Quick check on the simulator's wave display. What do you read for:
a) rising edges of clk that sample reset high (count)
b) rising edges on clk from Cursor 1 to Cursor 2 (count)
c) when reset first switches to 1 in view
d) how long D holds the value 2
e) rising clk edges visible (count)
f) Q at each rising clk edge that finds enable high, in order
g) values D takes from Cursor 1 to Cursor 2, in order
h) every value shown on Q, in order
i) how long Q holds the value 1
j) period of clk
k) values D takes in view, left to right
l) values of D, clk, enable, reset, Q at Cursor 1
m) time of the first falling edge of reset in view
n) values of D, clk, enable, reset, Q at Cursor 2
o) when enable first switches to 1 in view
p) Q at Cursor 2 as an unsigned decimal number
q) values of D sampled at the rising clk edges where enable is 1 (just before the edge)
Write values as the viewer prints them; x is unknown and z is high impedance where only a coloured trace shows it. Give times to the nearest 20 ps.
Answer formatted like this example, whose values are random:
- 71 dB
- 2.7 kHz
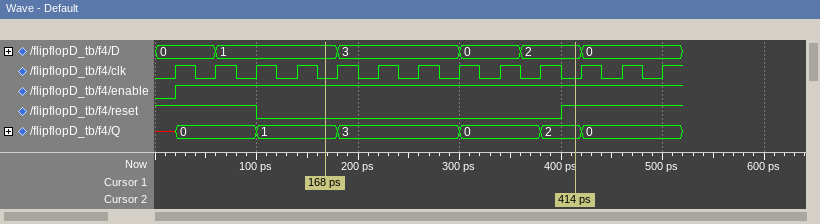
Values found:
- 6
- 6
- 400 ps
- 60 ps
- 13
- 0, 0, 1, 1, 3, 3, 3, 0, 0, 2, 0, 0
- 1, 3, 0, 2
- x, 0, 1, 3, 0, 2, 0
- 80 ps
- 40 ps
- 0, 1, 3, 0, 2, 0
- D=1, clk=0, enable=1, reset=0, Q=1
- 100 ps
- D=2, clk=0, enable=1, reset=1, Q=2
- 20 ps
- 2
- 0, 1, 1, 1, 3, 3, 3, 0, 2, 2, 0, 0
